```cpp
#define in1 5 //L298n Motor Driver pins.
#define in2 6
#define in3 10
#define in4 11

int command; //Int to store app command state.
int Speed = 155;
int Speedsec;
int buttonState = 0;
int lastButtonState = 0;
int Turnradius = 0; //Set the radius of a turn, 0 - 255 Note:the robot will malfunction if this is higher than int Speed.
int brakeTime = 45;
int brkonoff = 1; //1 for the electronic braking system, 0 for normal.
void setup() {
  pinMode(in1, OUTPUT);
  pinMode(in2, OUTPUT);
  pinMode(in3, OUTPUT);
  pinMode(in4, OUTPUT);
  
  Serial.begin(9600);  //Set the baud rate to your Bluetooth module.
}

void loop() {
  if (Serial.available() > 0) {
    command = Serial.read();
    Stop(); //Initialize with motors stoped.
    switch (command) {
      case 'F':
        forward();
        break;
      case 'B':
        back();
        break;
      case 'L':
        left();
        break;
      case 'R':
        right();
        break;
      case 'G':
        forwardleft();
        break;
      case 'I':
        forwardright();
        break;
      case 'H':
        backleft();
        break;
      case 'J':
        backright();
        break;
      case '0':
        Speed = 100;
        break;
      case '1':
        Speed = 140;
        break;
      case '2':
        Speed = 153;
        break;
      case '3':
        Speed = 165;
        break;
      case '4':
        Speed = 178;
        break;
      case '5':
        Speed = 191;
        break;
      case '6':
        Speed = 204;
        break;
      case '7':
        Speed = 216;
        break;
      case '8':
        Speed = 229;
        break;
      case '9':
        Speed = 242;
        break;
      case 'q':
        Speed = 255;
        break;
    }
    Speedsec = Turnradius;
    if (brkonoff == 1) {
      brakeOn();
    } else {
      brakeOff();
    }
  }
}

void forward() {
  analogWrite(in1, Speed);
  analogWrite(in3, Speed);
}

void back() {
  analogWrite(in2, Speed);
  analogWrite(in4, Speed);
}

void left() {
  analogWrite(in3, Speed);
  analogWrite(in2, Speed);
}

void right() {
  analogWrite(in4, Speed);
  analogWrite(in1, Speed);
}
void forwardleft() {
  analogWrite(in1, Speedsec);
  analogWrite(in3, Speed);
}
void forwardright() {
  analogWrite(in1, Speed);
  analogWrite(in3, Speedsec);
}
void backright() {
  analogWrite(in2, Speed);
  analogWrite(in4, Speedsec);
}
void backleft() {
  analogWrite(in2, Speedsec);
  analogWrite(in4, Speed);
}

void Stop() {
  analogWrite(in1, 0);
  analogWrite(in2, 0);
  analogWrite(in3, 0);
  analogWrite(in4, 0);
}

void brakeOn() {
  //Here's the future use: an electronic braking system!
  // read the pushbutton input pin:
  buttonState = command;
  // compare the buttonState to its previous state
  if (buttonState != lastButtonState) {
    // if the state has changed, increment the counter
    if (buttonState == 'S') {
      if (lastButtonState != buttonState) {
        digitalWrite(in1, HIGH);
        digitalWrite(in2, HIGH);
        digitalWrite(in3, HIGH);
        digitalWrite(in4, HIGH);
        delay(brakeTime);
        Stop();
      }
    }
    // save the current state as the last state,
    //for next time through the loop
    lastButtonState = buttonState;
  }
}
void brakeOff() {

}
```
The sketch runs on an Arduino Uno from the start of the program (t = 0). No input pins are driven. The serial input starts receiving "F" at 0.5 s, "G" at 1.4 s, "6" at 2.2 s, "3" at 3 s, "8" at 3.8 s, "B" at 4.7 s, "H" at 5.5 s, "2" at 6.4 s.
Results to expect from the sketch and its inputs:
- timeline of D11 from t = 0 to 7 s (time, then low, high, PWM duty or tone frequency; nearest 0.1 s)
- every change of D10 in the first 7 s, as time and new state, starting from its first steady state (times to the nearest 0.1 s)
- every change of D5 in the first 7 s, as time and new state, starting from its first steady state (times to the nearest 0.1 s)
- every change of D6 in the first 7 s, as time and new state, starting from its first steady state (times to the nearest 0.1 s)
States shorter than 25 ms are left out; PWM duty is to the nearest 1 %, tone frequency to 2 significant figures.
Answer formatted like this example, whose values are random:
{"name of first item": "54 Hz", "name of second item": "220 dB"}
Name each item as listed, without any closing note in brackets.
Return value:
{"timeline of D11 from t = 0 to 7 s": "0 s low; 4.7 s PWM 90 %; 6.4 s low", "every change of D10 in the first 7 s, as time and new state, starting from its first steady state": "0 s low; 0.5 s PWM 61 %; 2.2 s low", "every change of D5 in the first 7 s, as time and new state, starting from its first steady state": "0 s low; 0.5 s PWM 61 %; 1.4 s low", "every change of D6 in the first 7 s, as time and new state, starting from its first steady state": "0 s low; 4.7 s PWM 90 %; 5.5 s low"}
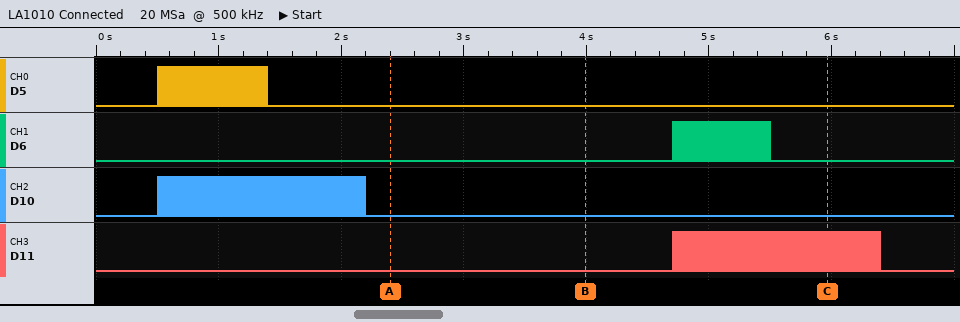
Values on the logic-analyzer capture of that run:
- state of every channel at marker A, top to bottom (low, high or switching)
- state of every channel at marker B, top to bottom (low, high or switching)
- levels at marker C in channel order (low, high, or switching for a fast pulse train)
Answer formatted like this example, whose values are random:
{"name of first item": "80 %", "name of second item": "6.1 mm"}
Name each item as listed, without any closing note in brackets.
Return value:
{"state of every channel at marker A, top to bottom": "D5 low, D6 low, D10 low, D11 low", "state of every channel at marker B, top to bottom": "D5 low, D6 low, D10 low, D11 low", "levels at marker C in channel order": "D5 low, D6 low, D10 low, D11 switching"}
